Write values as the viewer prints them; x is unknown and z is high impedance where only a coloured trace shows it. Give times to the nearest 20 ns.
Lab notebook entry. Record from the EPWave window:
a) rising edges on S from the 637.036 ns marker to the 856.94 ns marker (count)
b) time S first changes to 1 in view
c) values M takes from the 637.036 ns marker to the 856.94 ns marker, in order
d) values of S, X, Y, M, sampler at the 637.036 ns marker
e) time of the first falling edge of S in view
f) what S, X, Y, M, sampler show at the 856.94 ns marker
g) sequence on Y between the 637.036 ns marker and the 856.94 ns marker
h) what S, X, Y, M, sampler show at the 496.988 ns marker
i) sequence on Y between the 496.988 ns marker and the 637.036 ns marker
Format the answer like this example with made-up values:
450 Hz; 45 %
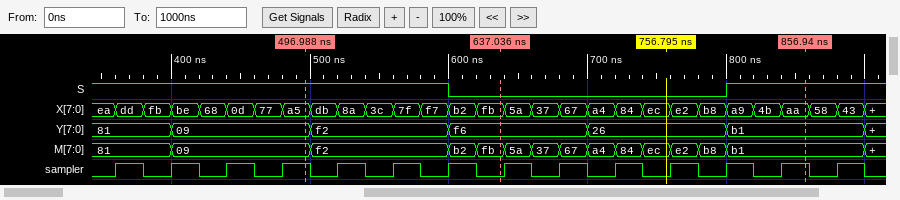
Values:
1; 800 ns; fb, 5a, 37, 67, a4, 84, ec, e2, b8, b1; S=0, X=fb, Y=f6, M=fb, sampler=0; 600 ns; S=1, X=aa, Y=b1, M=b1, sampler=1; f6, 26, b1; S=1, X=a5, Y=09, M=09, sampler=1; 09, f2, f6
